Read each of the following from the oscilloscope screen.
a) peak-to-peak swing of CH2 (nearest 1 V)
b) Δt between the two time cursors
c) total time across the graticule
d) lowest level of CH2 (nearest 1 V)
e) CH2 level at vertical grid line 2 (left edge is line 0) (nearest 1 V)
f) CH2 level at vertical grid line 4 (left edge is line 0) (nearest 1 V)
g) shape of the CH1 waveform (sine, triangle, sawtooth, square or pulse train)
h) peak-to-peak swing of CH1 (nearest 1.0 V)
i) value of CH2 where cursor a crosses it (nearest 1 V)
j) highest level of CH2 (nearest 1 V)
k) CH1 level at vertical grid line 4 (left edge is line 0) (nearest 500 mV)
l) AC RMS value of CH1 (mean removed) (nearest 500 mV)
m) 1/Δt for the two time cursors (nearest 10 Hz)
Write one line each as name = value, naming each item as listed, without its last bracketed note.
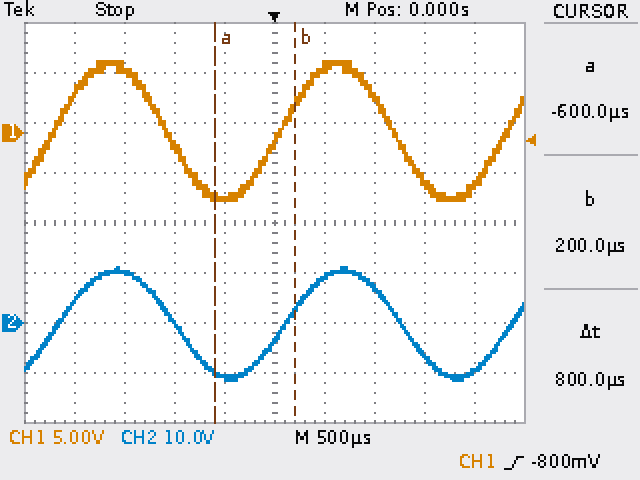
peak-to-peak swing of CH2 = 23 V
Δt between the two time cursors = 800 µs
total time across the graticule = 5 ms
lowest level of CH2 = -12 V
CH2 level at vertical grid line 2 (left edge is line 0) = 10 V
CH2 level at vertical grid line 4 (left edge is line 0) = -11 V
shape of the CH1 waveform = sine
peak-to-peak swing of CH1 = 14.0 V
value of CH2 where cursor a crosses it = -10 V
highest level of CH2 = 11 V
CH1 level at vertical grid line 4 (left edge is line 0) = -6.5 V
AC RMS value of CH1 (mean removed) = 5.0 V
1/Δt for the two time cursors = 1.25 kHz
